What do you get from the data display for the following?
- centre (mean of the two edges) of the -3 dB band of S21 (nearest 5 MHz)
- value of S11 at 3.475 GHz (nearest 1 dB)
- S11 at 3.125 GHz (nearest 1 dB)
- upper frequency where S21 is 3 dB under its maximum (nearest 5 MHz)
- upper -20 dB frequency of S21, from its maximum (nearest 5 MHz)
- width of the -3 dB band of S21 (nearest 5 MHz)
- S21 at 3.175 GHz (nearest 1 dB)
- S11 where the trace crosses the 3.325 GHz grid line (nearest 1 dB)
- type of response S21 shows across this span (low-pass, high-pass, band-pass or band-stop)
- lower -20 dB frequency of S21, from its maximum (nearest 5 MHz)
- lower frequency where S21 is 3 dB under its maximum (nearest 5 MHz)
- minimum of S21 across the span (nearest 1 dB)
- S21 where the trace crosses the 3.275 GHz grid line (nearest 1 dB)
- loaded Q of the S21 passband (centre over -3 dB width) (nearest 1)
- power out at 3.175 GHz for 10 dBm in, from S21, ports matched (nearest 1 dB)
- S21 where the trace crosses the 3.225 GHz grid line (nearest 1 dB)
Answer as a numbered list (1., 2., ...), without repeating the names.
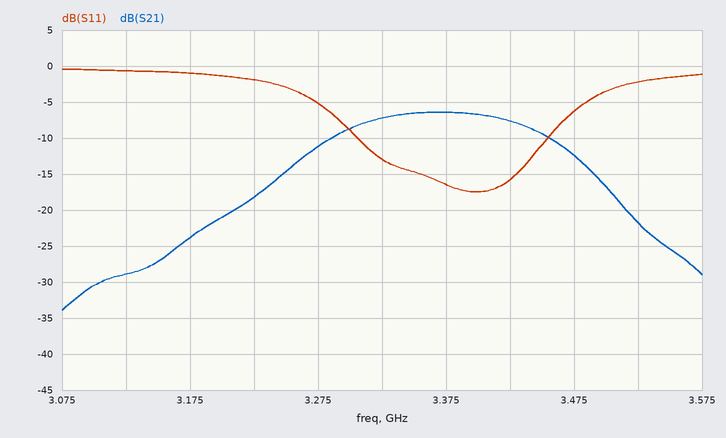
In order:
1. 3.370 GHz
2. -6 dB
3. -1 dB
4. 3.450 GHz
5. 3.560 GHz
6. 160 MHz
7. -24 dB
8. -13 dB
9. band-pass
10. 3.155 GHz
11. 3.290 GHz
12. -34 dB
13. -11 dB
14. 21
15. -14 dBm
16. -18 dB
